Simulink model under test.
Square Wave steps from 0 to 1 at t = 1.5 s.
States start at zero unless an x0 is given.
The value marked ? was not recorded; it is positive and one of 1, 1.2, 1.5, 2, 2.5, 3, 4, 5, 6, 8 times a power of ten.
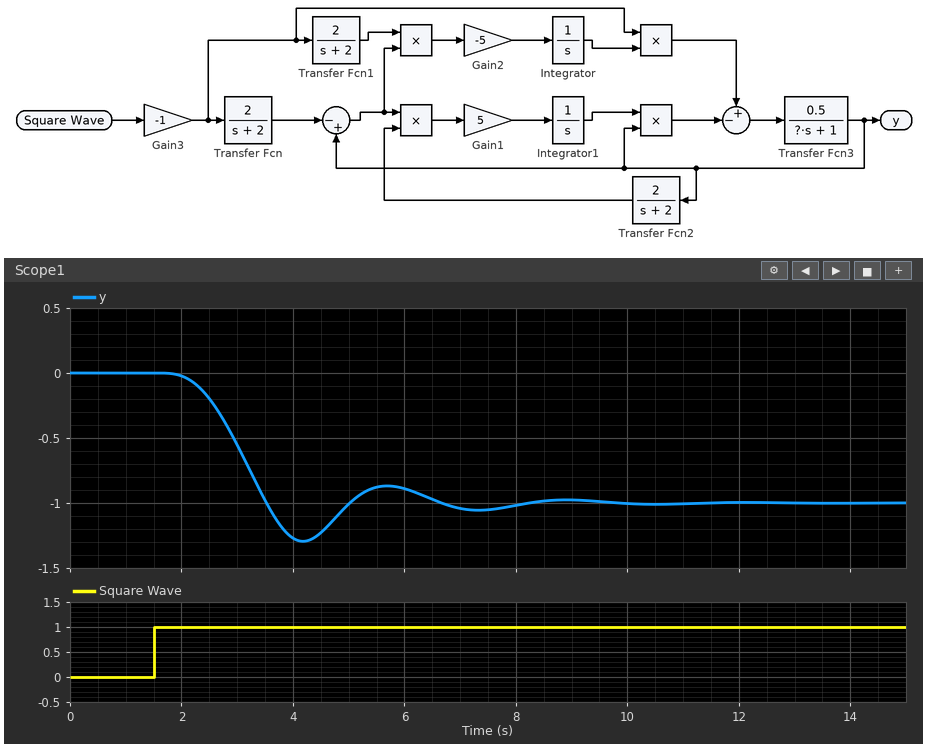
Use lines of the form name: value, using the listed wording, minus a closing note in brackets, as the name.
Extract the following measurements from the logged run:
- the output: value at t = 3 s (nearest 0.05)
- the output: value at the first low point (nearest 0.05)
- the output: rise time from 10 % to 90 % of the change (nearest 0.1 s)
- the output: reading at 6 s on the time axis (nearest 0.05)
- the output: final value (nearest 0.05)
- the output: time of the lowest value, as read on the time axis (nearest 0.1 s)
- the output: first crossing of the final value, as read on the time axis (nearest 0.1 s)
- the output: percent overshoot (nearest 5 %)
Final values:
the output: value at t = 3 s: -0.55
the output: value at the first low point: -1.30
the output: rise time from 10 % to 90 % of the change: 1.1 s
the output: reading at 6 s on the time axis: -0.90
the output: final value: -1.00
the output: time of the lowest value, as read on the time axis: 4.2 s
the output: first crossing of the final value, as read on the time axis: 3.5 s
the output: percent overshoot: 30 %
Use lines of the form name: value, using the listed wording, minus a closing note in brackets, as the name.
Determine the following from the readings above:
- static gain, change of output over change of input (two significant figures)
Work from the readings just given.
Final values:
static gain, change of output over change of input: -1.0
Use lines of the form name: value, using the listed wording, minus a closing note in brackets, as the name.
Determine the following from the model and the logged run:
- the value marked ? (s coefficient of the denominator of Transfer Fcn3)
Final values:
the value marked ?: 1.2
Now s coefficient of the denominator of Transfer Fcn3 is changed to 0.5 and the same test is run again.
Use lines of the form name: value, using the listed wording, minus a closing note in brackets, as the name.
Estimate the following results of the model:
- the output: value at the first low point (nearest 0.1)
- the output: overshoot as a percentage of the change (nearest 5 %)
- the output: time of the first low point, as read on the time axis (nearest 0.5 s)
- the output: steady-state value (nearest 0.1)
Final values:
the output: value at the first low point: -1.1
the output: overshoot as a percentage of the change: 15 %
the output: time of the first low point, as read on the time axis: 3.5 s
the output: steady-state value: -1.0
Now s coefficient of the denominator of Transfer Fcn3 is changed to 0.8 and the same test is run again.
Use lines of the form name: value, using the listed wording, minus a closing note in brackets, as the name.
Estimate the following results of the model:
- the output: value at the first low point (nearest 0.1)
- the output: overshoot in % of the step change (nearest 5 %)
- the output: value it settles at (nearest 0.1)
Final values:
the output: value at the first low point: -1.2
the output: overshoot in % of the step change: 20 %
the output: value it settles at: -1.0
